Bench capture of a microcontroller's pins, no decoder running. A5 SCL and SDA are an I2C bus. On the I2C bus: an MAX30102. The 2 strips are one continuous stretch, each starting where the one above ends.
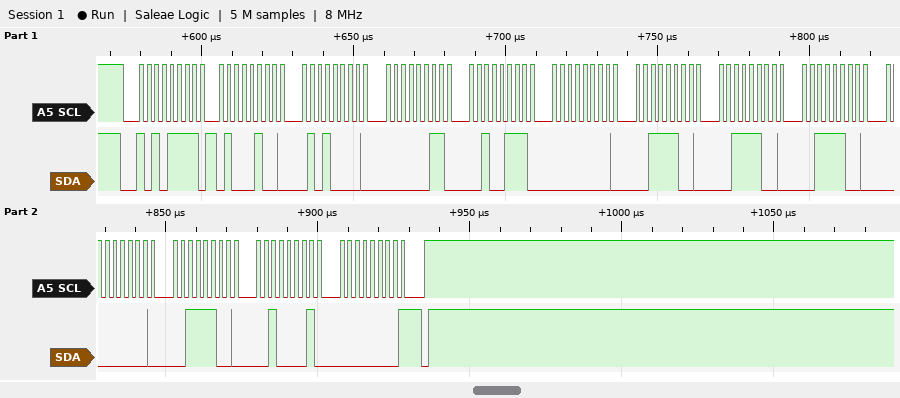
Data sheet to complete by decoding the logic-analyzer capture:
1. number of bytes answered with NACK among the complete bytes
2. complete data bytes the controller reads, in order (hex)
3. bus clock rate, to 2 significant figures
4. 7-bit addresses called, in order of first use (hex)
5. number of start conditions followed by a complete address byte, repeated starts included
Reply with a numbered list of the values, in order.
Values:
1. 1
2. 44 50 03 27 00 3C 3C 3C 00 3C 21 00
3. 400 kHz
4. 0x57
5. 1
